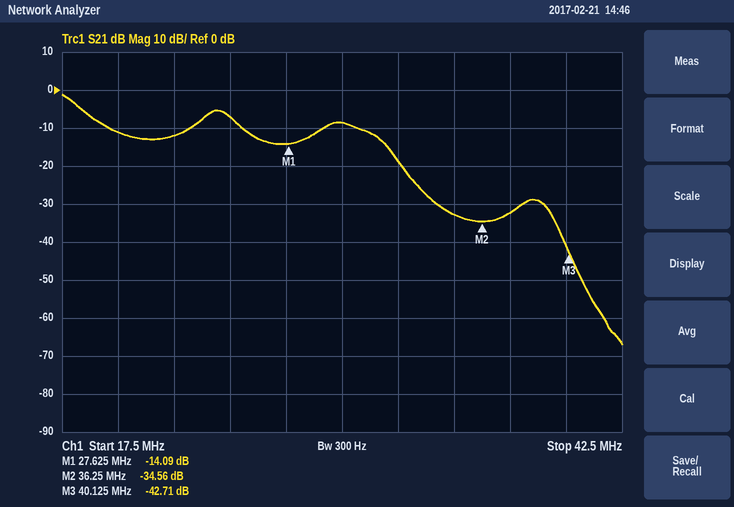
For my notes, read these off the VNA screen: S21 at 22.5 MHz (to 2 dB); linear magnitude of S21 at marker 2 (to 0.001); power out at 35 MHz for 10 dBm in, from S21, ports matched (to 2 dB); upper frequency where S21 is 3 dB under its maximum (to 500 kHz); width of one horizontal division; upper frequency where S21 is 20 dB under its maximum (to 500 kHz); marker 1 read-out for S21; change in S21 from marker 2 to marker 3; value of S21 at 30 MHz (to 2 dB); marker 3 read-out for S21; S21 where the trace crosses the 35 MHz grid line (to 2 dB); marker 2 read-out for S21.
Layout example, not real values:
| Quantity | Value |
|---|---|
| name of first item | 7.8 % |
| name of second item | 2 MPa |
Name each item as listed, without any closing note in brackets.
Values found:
| Quantity | Value |
|---|---|
| S21 at 22.5 MHz | -12 dB |
| linear magnitude of S21 at marker 2 | 0.019 |
| power out at 35 MHz for 10 dBm in, from S21, ports matched | -22 dBm |
| upper frequency where S21 is 3 dB under its maximum | 18.0 MHz |
| width of one horizontal division | 2.5 MHz |
| upper frequency where S21 is 20 dB under its maximum | 33.0 MHz |
| marker 1 read-out for S21 | -14.09 dB |
| change in S21 from marker 2 to marker 3 | -8.15 dB |
| value of S21 at 30 MHz | -8 dB |
| marker 3 read-out for S21 | -42.71 dB |
| S21 where the trace crosses the 35 MHz grid line | -32 dB |
| marker 2 read-out for S21 | -34.56 dB |
